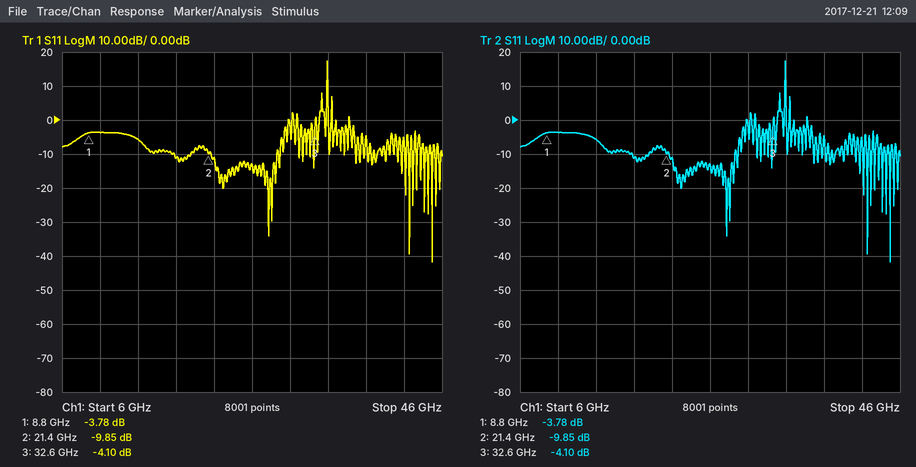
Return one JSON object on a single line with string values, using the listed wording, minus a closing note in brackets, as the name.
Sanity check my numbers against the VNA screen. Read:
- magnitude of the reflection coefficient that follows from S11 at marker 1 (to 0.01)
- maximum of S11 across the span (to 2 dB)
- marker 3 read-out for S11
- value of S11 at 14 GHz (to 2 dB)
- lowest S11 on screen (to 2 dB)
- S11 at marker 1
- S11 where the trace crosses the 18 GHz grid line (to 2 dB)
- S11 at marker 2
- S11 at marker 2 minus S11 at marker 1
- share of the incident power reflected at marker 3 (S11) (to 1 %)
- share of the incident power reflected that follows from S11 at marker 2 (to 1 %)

{"magnitude of the reflection coefficient that follows from S11 at marker 1": "0.65", "maximum of S11 across the span": "18 dB", "marker 3 read-out for S11": "-4.10 dB", "value of S11 at 14 GHz": "-6 dB", "lowest S11 on screen": "-42 dB", "S11 at marker 1": "-3.78 dB", "S11 where the trace crosses the 18 GHz grid line": "-12 dB", "S11 at marker 2": "-9.85 dB", "S11 at marker 2 minus S11 at marker 1": "-6.07 dB", "share of the incident power reflected at marker 3 (S11)": "39 %", "share of the incident power reflected that follows from S11 at marker 2": "10 %"}
